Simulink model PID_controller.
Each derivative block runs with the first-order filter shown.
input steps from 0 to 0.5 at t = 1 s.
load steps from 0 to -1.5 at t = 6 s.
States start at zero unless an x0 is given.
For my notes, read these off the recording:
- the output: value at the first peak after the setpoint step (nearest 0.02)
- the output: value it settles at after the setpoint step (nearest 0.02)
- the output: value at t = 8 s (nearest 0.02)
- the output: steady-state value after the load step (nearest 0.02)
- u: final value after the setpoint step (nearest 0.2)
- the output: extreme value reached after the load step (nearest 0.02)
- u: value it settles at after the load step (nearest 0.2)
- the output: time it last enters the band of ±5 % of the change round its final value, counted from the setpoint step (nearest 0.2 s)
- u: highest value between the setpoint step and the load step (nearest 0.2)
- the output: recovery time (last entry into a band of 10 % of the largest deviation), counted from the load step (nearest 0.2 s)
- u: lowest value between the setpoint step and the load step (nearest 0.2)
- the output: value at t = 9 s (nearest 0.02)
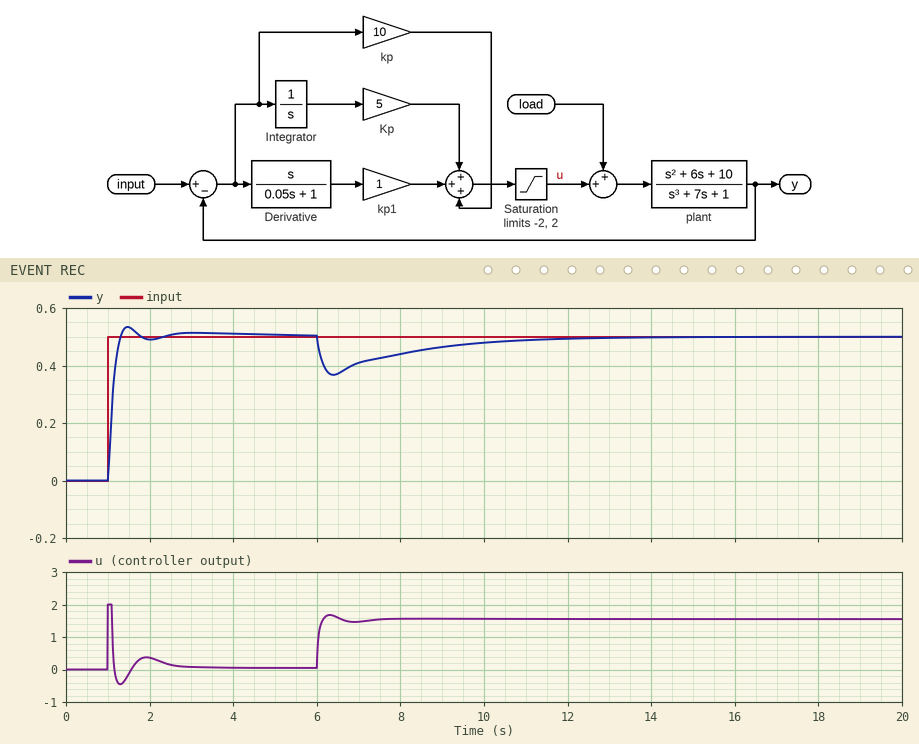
0.54
0.50
0.44
0.50
0.0
0.36
1.6
0.6 s
2.0
4.8 s
-0.4
0.46
